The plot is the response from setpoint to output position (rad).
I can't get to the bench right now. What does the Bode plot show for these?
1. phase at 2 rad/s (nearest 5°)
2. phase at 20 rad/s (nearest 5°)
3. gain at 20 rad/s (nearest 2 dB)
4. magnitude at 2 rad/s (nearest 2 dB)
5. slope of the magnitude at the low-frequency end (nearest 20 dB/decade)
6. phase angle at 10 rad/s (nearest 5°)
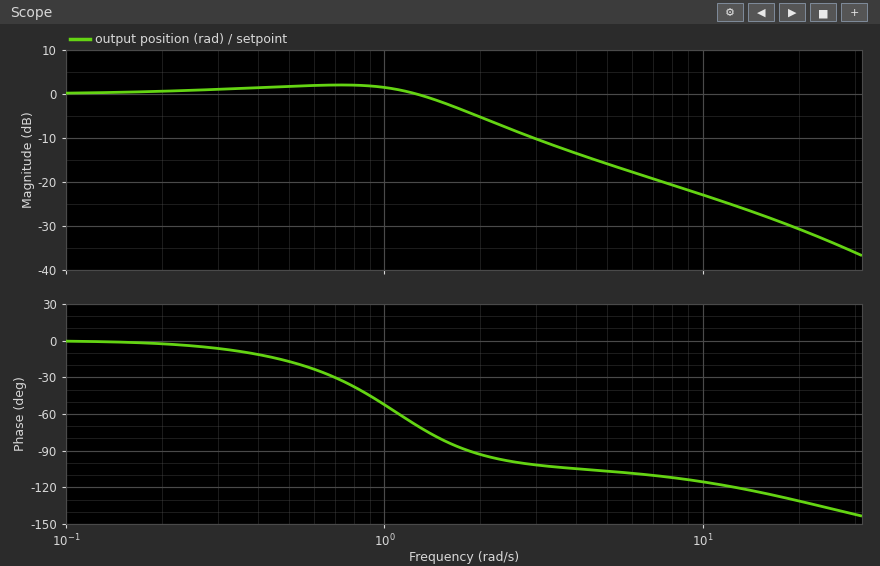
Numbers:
-95°
-130°
-30 dB
-6 dB
0 dB/decade
-115°
